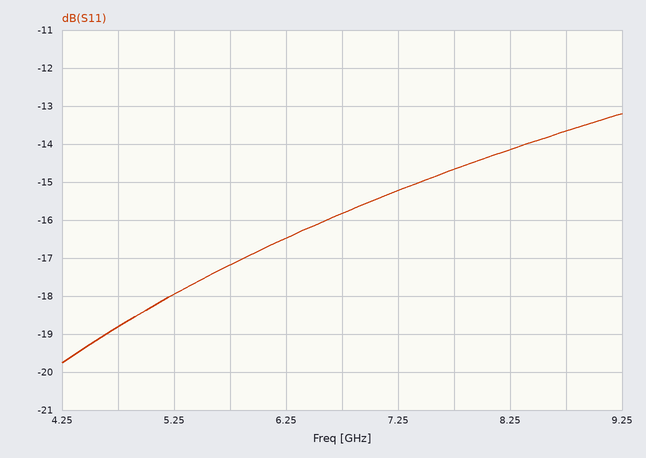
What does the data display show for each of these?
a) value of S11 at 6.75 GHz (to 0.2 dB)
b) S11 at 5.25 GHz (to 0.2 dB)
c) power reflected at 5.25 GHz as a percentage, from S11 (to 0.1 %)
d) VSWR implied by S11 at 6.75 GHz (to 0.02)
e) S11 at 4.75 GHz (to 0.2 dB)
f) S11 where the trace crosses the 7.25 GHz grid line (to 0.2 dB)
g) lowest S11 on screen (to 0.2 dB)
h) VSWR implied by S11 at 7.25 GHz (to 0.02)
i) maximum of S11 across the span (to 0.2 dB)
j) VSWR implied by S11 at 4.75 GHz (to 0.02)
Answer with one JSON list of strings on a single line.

["-15.8 dB", "-18.0 dB", "1.6 %", "1.38", "-18.8 dB", "-15.2 dB", "-19.8 dB", "1.42", "-13.2 dB", "1.26"]
